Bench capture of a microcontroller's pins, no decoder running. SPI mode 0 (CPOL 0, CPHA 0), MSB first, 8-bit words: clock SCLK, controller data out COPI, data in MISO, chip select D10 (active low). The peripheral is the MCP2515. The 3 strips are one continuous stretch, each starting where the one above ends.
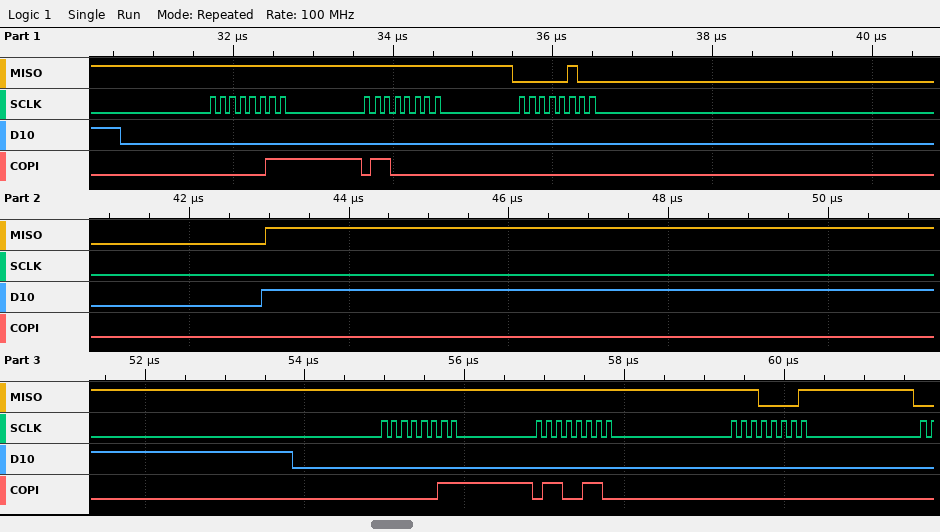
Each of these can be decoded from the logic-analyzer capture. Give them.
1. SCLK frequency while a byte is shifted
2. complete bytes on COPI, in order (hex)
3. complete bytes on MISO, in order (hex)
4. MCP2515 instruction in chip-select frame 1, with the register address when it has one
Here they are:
8 MHz
03 60 00 03 66 00
FF FF 04 FF FF E1
READ 0x60
